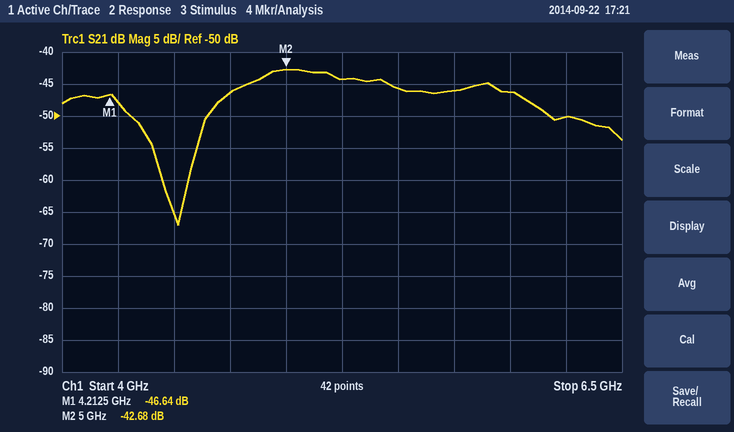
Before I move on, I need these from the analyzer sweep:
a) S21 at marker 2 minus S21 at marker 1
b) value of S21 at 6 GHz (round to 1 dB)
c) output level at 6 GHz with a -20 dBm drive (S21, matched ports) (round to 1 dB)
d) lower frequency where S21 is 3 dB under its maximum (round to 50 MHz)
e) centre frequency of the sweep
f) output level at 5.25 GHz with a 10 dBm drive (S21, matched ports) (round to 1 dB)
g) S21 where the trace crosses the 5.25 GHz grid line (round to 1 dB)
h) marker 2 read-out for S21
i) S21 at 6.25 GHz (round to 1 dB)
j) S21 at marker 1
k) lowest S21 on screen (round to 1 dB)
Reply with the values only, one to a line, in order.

3.96 dB
-46 dB
-66 dBm
4.80 GHz
5.25 GHz
-34 dBm
-44 dB
-42.68 dB
-50 dB
-46.64 dB
-67 dB
